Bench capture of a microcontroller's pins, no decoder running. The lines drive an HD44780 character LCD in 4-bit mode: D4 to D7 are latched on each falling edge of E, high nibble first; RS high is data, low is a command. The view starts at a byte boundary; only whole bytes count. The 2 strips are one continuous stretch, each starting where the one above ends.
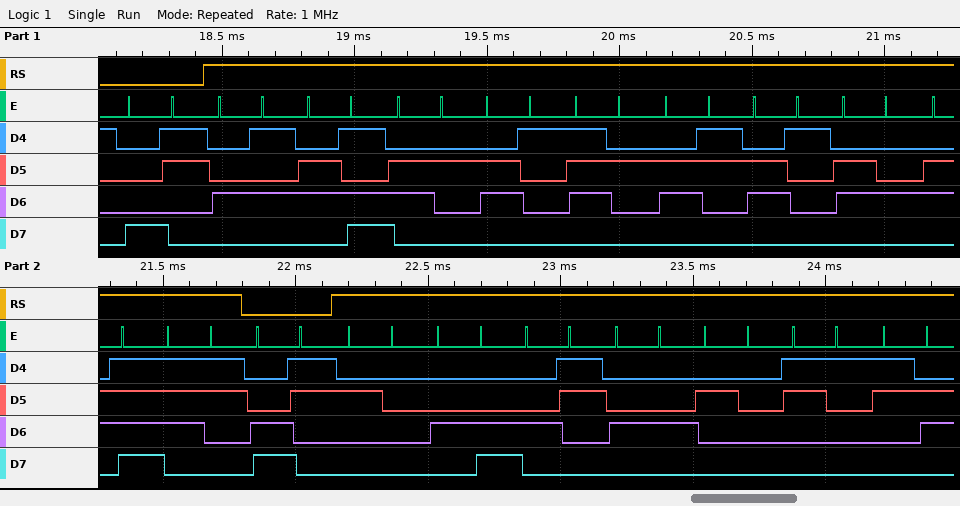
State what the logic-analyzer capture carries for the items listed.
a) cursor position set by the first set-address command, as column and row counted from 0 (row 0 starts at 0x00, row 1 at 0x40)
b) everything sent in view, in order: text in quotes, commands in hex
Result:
column 3, row 0
0x83 "Embarcados" 0xC3 " LCD 16"
